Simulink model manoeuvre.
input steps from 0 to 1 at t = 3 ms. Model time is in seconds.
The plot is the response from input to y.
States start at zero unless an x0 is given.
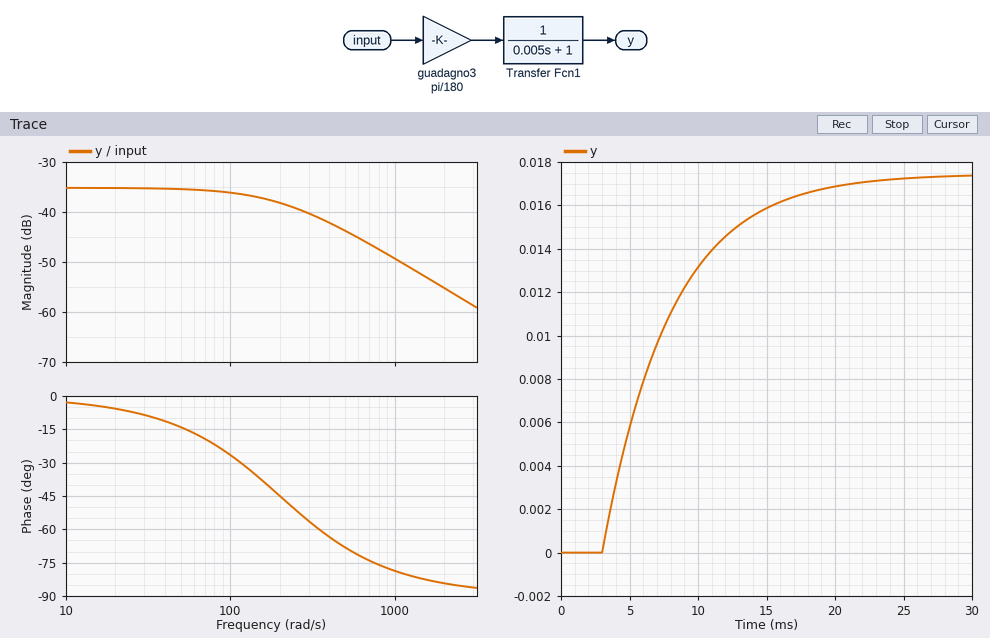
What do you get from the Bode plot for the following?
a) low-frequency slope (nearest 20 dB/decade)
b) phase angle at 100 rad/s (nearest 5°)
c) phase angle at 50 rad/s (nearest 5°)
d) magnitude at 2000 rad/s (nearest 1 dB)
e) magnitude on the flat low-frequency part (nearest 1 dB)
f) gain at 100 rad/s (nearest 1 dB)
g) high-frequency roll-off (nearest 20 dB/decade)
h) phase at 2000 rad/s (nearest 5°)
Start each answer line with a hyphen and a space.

- 0 dB/decade
- -25°
- -15°
- -55 dB
- -35 dB
- -36 dB
- -20 dB/decade
- -85°
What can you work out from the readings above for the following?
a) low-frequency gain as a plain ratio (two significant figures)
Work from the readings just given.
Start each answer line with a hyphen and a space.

- 0.018
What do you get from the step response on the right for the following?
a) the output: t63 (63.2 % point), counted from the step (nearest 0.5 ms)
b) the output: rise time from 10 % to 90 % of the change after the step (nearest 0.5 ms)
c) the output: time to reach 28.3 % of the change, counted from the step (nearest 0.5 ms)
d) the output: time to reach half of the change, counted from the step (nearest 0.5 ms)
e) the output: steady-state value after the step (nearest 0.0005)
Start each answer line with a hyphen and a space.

- 5.0 ms
- 11.0 ms
- 1.5 ms
- 3.5 ms
- 0.0175
